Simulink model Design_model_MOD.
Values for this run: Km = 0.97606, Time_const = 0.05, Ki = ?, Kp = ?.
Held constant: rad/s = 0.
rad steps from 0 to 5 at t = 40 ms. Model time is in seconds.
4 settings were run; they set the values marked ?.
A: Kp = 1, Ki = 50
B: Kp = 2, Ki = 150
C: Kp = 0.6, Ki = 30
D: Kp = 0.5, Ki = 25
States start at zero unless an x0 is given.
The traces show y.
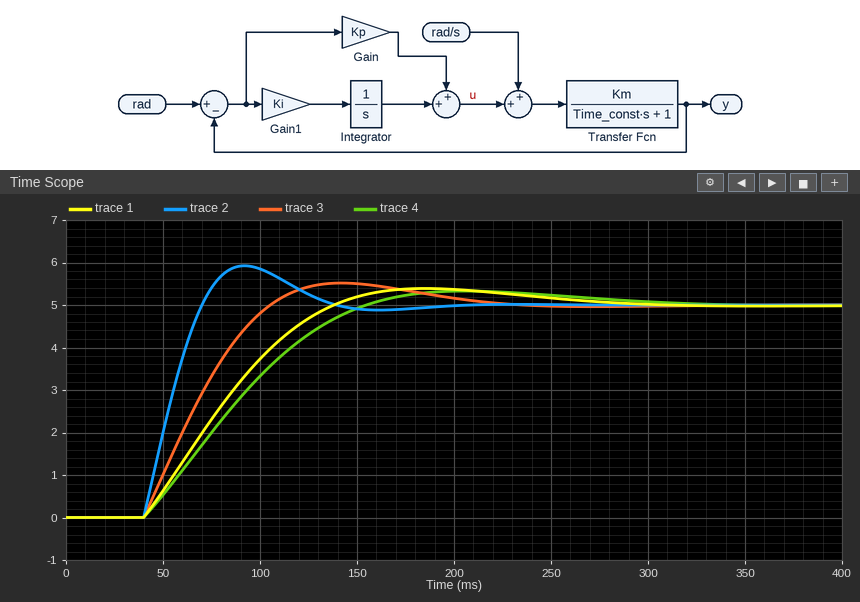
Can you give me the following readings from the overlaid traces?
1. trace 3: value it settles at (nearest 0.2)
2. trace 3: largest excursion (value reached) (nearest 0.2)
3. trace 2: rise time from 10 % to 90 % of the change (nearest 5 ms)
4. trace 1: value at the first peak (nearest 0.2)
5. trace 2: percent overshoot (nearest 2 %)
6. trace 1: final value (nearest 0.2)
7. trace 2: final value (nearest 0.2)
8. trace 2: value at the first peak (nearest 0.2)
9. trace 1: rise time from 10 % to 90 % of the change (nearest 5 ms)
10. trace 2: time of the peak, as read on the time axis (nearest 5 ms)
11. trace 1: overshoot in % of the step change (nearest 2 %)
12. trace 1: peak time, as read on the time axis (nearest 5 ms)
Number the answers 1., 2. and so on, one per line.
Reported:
1. 5.0
2. 5.6
3. 25 ms
4. 5.4
5. 18 %
6. 5.0
7. 5.0
8. 6.0
9. 70 ms
10. 90 ms
11. 8 %
12. 185 ms
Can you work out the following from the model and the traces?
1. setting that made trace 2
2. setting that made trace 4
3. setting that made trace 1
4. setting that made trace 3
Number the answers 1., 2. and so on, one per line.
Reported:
1. B
2. D
3. C
4. A
